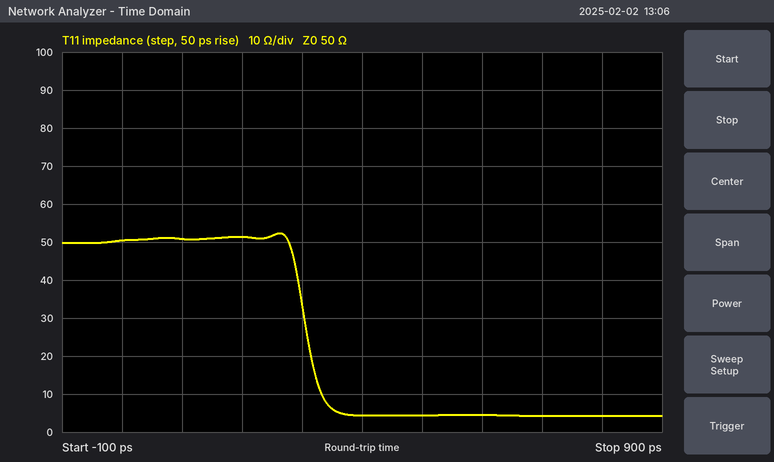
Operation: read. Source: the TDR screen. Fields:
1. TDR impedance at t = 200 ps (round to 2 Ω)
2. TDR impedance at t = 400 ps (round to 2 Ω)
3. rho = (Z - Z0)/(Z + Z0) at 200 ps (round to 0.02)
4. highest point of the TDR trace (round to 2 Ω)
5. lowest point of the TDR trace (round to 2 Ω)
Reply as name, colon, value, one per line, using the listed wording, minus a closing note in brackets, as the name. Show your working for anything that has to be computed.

TDR impedance at t = 200 ps: 52 Ω
TDR impedance at t = 400 ps: 4 Ω
rho = (Z - Z0)/(Z + Z0) at 200 ps: (52 − 50)/(52 + 50) ≈ +0.02
highest point of the TDR trace: 52 Ω
lowest point of the TDR trace: 4 Ω
